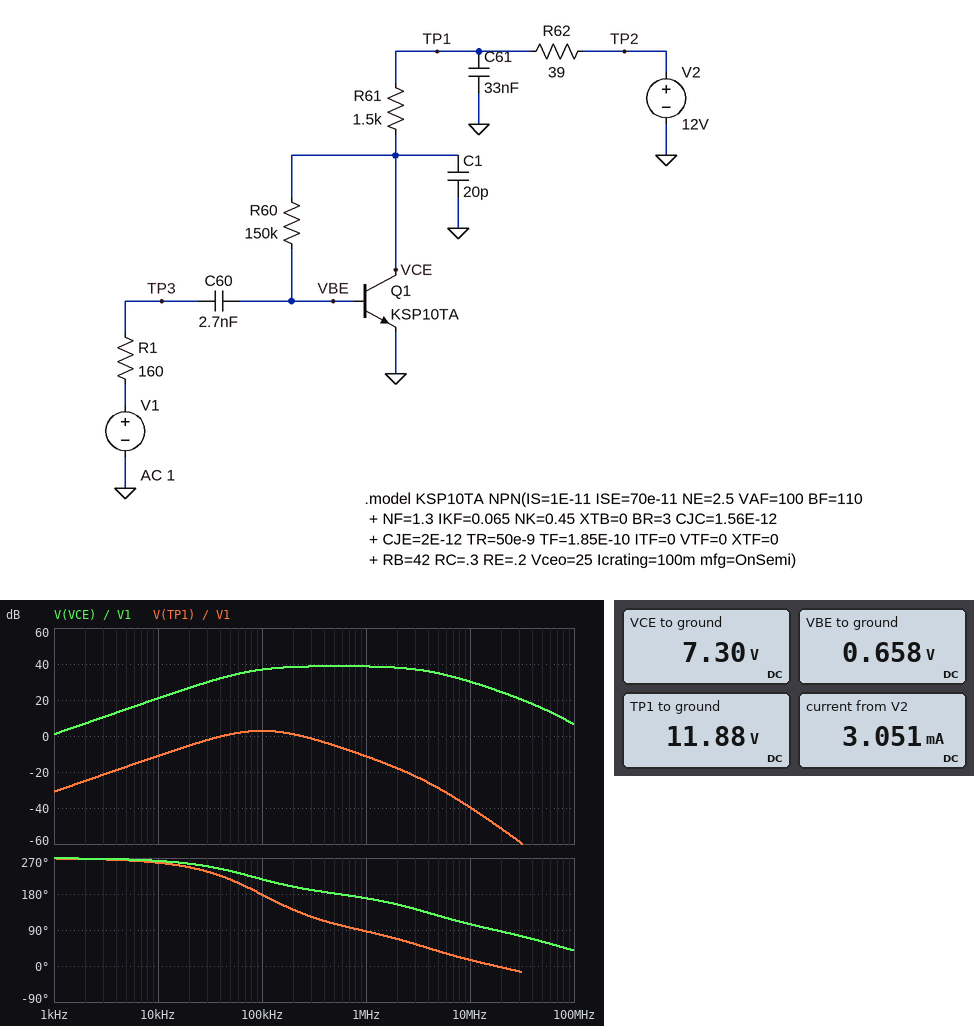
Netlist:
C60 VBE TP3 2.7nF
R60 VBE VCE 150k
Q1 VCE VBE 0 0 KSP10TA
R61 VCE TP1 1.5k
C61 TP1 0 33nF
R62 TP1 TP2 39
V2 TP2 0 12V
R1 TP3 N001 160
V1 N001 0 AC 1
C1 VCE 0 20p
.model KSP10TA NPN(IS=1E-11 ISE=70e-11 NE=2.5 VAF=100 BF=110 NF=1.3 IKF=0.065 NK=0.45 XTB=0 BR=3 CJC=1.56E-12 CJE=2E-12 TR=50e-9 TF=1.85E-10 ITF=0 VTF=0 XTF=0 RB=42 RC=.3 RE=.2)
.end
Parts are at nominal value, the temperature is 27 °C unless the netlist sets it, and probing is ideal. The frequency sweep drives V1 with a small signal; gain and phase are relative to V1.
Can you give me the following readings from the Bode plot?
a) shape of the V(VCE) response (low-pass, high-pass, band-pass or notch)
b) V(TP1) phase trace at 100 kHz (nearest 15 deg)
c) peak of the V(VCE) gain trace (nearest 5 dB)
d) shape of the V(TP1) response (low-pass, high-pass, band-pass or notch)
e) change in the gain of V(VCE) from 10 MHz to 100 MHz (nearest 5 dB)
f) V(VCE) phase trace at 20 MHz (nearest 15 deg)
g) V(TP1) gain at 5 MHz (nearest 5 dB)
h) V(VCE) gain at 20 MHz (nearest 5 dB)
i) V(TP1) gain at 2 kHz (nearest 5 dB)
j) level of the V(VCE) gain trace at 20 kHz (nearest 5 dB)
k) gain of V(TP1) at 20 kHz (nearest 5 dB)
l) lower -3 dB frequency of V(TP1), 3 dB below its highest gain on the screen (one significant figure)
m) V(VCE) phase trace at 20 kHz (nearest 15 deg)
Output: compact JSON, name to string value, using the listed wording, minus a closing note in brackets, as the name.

{"shape of the V(VCE) response": "band-pass", "V(TP1) phase trace at 100 kHz": "180 deg", "peak of the V(VCE) gain trace": "40 dB", "shape of the V(TP1) response": "band-pass", "change in the gain of V(VCE) from 10 MHz to 100 MHz": "-25 dB", "V(VCE) phase trace at 20 MHz": "90 deg", "V(TP1) gain at 5 MHz": "-30 dB", "V(VCE) gain at 20 MHz": "25 dB", "V(TP1) gain at 2 kHz": "-25 dB", "level of the V(VCE) gain trace at 20 kHz": "25 dB", "gain of V(TP1) at 20 kHz": "-5 dB", "lower -3 dB frequency of V(TP1), 3 dB below its highest gain on the screen": "40 kHz", "V(VCE) phase trace at 20 kHz": "255 deg"}
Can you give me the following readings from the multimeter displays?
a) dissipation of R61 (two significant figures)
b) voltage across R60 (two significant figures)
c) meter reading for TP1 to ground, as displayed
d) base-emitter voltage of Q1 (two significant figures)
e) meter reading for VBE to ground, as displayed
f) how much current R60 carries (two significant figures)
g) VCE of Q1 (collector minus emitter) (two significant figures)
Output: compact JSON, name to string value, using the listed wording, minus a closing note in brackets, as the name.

{"dissipation of R61": "14 mW", "voltage across R60": "6.6 V", "meter reading for TP1 to ground, as displayed": "11.88 V", "base-emitter voltage of Q1": "660 mV", "meter reading for VBE to ground, as displayed": "0.658 V", "how much current R60 carries": "44 µA", "VCE of Q1 (collector minus emitter)": "7.3 V"}
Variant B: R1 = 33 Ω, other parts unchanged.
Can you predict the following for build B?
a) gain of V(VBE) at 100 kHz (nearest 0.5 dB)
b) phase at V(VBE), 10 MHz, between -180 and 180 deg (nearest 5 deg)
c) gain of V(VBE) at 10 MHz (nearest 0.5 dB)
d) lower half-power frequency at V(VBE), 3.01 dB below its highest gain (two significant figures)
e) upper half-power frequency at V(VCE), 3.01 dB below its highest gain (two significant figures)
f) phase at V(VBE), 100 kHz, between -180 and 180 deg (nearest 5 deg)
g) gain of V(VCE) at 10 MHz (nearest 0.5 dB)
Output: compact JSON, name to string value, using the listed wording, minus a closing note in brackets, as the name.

{"gain of V(VBE) at 100 kHz": "-3.5 dB", "phase at V(VBE), 10 MHz, between -180 and 180 deg": "0 deg", "gain of V(VBE) at 10 MHz": "-1.0 dB", "lower half-power frequency at V(VBE), 3.01 dB below its highest gain": "96 kHz", "upper half-power frequency at V(VCE), 3.01 dB below its highest gain": "4.8 MHz", "phase at V(VBE), 100 kHz, between -180 and 180 deg": "45 deg", "gain of V(VCE) at 10 MHz": "33.0 dB"}
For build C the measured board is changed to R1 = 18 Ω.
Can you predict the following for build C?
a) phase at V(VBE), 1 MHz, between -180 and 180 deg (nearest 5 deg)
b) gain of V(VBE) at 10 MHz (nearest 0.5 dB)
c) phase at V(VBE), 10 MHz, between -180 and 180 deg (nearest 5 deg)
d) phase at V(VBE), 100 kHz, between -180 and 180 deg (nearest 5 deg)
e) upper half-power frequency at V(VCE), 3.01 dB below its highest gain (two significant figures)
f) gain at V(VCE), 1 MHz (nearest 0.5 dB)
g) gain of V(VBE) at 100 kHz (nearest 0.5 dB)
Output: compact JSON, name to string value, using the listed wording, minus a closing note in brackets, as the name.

{"phase at V(VBE), 1 MHz, between -180 and 180 deg": "5 deg", "gain of V(VBE) at 10 MHz": "-0.5 dB", "phase at V(VBE), 10 MHz, between -180 and 180 deg": "0 deg", "phase at V(VBE), 100 kHz, between -180 and 180 deg": "45 deg", "upper half-power frequency at V(VCE), 3.01 dB below its highest gain": "4.9 MHz", "gain at V(VCE), 1 MHz": "40.5 dB", "gain of V(VBE) at 100 kHz": "-3.5 dB"}
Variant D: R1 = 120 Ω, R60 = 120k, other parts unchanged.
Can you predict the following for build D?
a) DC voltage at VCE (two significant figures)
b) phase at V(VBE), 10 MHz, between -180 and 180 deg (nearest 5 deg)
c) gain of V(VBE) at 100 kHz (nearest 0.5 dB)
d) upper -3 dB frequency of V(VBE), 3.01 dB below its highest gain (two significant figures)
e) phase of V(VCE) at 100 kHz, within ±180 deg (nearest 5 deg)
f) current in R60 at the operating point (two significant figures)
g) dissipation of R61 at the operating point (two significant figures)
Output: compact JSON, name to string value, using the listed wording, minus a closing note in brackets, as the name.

{"DC voltage at VCE": "6.6 V", "phase at V(VBE), 10 MHz, between -180 and 180 deg": "-5 deg", "gain of V(VBE) at 100 kHz": "-5.5 dB", "upper -3 dB frequency of V(VBE), 3.01 dB below its highest gain": "67 MHz", "phase of V(VCE) at 100 kHz, within ±180 deg": "-135 deg", "current in R60 at the operating point": "50 µA", "dissipation of R61 at the operating point": "18 mW"}
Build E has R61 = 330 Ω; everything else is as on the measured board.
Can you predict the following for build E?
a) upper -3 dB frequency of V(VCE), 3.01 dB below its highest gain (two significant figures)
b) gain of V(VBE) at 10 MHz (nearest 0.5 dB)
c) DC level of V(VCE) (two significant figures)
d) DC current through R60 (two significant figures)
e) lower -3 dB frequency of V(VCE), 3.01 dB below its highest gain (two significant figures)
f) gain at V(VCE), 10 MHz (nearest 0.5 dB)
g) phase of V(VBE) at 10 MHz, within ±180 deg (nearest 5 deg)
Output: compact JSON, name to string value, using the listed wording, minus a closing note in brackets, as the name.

{"upper -3 dB frequency of V(VCE), 3.01 dB below its highest gain": "13 MHz", "gain of V(VBE) at 10 MHz": "-3.5 dB", "DC level of V(VCE)": "10 V", "DC current through R60": "64 µA", "lower -3 dB frequency of V(VCE), 3.01 dB below its highest gain": "67 kHz", "gain at V(VCE), 10 MHz": "27.5 dB", "phase of V(VBE) at 10 MHz, within ±180 deg": "-15 deg"}
